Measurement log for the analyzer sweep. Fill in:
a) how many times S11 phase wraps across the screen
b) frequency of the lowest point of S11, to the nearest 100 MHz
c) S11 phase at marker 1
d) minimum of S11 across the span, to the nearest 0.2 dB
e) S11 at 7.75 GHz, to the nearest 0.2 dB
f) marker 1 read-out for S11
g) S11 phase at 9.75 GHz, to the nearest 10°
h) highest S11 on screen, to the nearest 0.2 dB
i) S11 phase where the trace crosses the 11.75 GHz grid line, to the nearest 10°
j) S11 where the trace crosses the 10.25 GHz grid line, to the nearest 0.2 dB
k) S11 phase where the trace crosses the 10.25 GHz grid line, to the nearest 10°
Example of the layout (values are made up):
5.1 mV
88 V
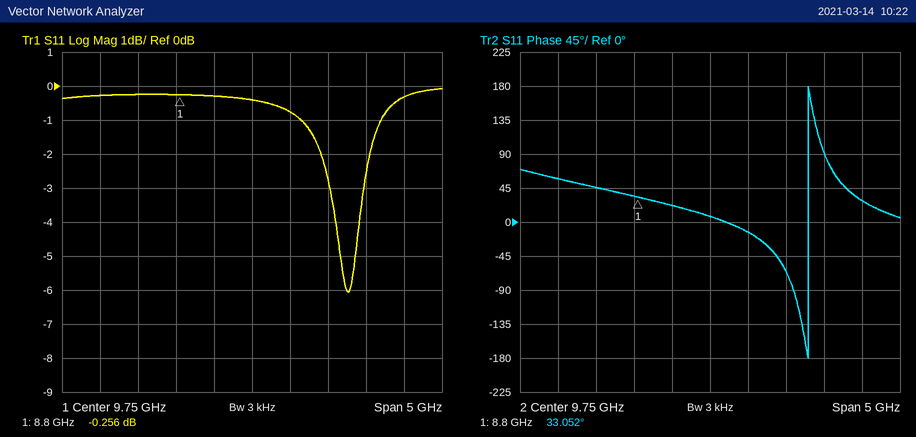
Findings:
1
11.0 GHz
33.052°
-6.0 dB
-0.2 dB
-0.256 dB
10°
0.0 dB
30°
-0.8 dB
-10°
